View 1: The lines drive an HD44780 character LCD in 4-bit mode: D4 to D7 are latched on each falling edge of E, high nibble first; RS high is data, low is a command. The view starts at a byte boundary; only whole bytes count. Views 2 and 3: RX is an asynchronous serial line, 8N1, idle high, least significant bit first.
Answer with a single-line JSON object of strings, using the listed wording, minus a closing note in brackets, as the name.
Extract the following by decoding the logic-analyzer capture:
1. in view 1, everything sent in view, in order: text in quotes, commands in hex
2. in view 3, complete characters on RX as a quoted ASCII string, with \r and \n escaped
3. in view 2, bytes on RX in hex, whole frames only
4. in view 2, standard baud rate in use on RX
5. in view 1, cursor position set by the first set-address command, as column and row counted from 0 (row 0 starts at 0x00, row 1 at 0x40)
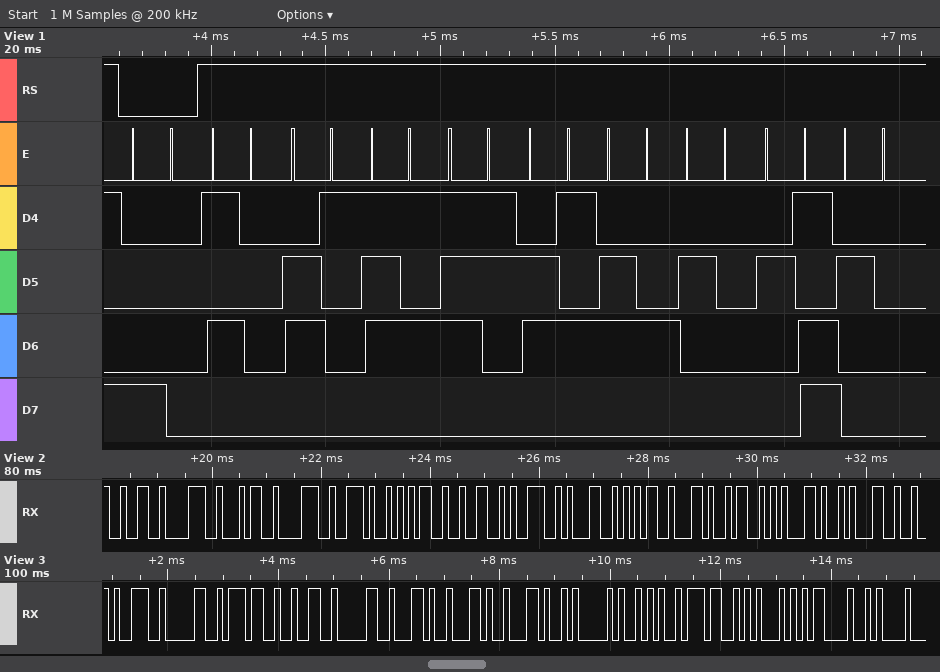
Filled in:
{"in view 1, everything sent in view, in order: text in quotes, commands in hex": "0x80 \"Paused - \"", "in view 3, complete characters on RX as a quoted ASCII string, with \\r and \\n escaped": "\"90720,,,A*7E\\r\\n\"", "in view 2, bytes on RX in hex, whole frames only": "32 38 34 38 2E 35 32 39 31 35 2C 53 2C 31", "in view 2, standard baud rate in use on RX": "9600 baud", "in view 1, cursor position set by the first set-address command, as column and row counted from 0": "column 0, row 0"}
